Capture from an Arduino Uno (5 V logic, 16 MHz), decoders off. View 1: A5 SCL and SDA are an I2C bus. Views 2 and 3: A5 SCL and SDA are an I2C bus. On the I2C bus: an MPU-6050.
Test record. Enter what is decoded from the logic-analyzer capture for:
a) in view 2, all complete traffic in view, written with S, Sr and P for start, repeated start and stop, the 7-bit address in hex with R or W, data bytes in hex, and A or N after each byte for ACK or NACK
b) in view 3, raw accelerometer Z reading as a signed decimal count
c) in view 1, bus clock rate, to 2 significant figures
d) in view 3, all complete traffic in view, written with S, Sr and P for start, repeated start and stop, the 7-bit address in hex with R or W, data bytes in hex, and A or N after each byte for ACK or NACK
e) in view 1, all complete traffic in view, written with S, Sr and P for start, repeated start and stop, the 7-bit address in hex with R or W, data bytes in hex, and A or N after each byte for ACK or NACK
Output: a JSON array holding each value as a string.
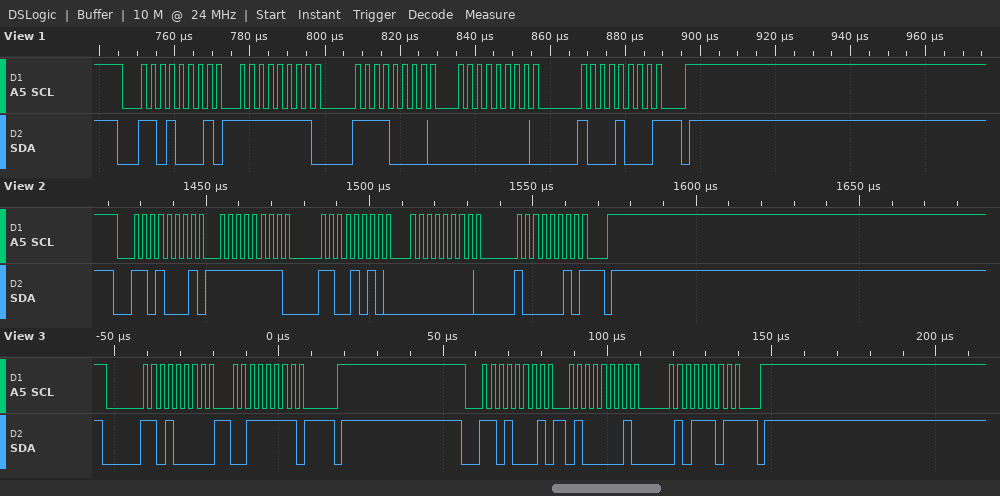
["S 68R A FF A CA A 00 A 82 N P", "16733", "400 kHz", "S 68W A 3F A P S 68R A 41 A 5D N P", "S 68R A FF A F0 A 00 A 88 N P"]
